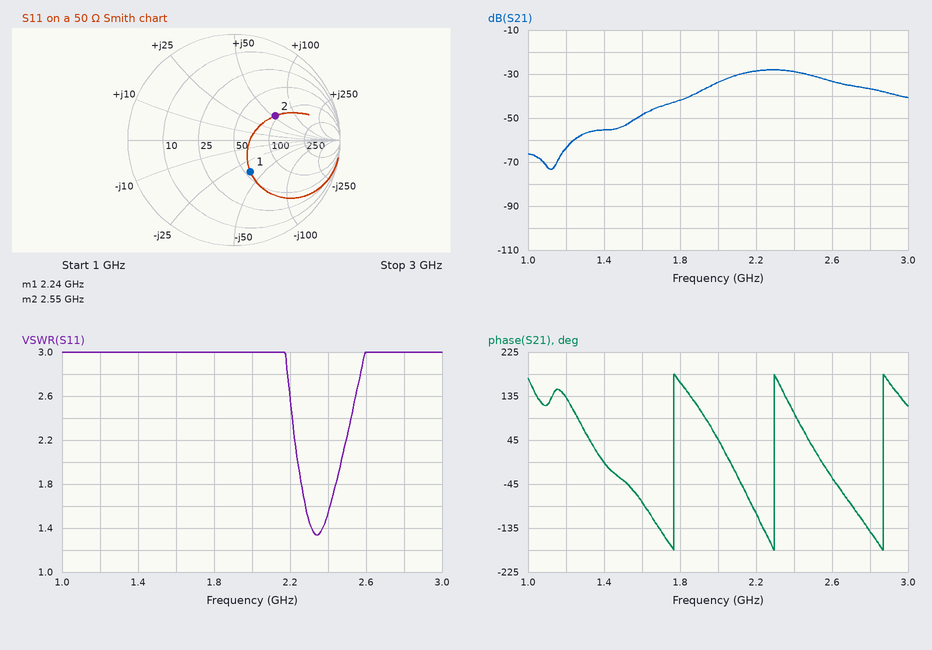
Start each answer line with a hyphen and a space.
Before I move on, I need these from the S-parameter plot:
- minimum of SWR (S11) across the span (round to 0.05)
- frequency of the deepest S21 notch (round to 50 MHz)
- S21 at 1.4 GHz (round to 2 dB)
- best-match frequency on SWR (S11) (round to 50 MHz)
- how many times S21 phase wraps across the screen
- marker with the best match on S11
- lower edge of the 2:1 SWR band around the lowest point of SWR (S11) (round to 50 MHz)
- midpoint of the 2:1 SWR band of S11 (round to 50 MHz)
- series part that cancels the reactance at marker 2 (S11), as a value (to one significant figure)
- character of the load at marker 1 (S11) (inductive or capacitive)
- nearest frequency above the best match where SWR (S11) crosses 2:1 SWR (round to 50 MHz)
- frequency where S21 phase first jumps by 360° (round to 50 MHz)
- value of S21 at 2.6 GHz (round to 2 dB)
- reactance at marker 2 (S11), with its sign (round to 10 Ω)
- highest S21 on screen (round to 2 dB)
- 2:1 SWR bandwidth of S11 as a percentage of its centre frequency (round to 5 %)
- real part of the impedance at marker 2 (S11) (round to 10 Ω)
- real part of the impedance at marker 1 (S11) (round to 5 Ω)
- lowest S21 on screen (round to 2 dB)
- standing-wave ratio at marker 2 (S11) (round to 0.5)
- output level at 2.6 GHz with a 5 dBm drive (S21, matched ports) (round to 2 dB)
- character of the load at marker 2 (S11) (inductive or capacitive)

- 1.35
- 1.10 GHz
- -56 dB
- 2.35 GHz
- 3
- marker 1
- 2.25 GHz
- 2.35 GHz
- 1 pF
- capacitive
- 2.45 GHz
- 1.75 GHz
- -34 dB
- +50 Ω
- -28 dB
- 10 %
- 90 Ω
- 55 Ω
- -74 dB
- 2.5
- -28 dBm
- inductive
